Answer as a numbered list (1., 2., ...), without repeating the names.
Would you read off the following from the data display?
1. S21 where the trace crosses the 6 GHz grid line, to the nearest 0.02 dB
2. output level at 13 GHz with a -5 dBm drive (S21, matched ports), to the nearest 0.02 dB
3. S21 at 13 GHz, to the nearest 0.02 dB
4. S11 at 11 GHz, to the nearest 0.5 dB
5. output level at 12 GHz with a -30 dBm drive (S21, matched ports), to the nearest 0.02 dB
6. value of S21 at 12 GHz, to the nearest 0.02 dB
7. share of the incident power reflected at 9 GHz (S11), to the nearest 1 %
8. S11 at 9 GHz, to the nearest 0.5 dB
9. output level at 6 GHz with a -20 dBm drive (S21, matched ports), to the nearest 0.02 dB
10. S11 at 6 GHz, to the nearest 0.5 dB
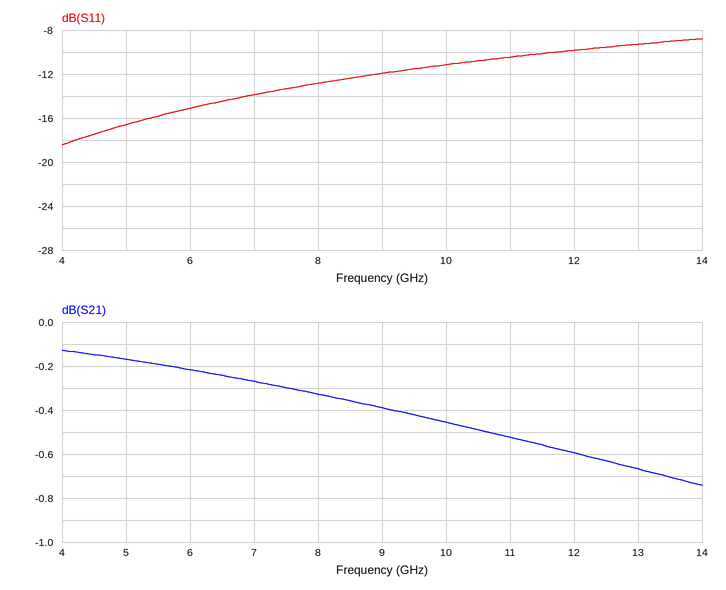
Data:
1. -0.22 dB
2. -5.66 dBm
3. -0.66 dB
4. -10.5 dB
5. -30.60 dBm
6. -0.60 dB
7. 6 %
8. -12.0 dB
9. -20.22 dBm
10. -15.0 dB
